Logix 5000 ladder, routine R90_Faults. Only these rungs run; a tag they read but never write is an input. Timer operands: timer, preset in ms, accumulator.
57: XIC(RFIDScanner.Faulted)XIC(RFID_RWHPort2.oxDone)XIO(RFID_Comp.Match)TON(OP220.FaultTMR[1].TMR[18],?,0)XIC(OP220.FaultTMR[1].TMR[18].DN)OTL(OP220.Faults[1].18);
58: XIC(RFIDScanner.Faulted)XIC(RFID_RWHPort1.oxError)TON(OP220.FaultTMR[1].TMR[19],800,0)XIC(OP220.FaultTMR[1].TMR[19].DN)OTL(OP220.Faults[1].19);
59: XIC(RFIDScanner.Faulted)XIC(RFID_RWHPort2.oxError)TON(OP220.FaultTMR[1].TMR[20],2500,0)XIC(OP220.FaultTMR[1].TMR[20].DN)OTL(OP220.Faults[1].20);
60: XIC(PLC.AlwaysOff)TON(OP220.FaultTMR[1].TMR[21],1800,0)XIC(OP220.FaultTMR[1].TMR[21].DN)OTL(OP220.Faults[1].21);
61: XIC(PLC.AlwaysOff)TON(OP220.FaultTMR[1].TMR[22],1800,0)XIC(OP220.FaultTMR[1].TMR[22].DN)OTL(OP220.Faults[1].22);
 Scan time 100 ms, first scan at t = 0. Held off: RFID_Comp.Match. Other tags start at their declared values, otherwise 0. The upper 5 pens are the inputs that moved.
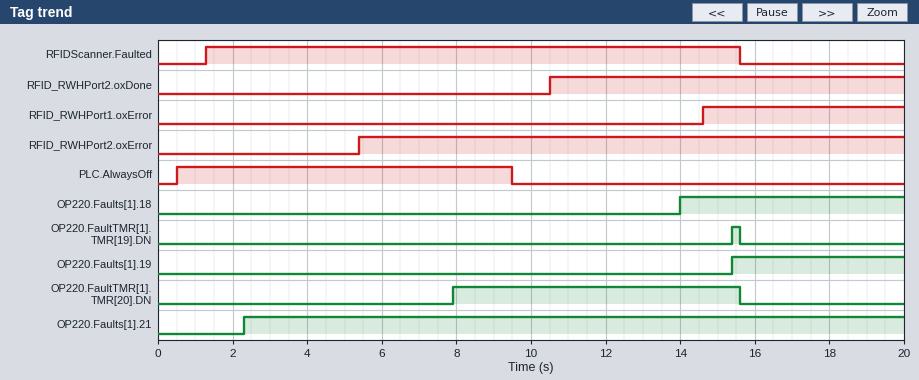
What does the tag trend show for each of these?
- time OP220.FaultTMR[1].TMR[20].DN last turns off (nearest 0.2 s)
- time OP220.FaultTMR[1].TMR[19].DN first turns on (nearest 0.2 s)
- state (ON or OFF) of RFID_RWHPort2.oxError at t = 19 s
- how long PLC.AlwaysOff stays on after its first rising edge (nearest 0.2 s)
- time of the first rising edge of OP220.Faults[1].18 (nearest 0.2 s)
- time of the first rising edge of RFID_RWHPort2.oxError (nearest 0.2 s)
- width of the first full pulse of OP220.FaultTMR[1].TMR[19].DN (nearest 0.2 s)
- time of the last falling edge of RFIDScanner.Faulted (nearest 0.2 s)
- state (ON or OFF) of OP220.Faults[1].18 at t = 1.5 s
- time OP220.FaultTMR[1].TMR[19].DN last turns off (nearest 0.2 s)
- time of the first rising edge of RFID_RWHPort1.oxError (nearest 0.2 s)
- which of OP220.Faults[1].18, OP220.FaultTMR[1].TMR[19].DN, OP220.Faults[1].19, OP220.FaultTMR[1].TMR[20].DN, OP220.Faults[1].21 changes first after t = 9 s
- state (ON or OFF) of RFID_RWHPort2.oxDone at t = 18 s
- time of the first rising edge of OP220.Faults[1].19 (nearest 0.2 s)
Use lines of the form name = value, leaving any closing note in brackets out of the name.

time OP220.FaultTMR[1].TMR[20].DN last turns off = 15.6 s
time OP220.FaultTMR[1].TMR[19].DN first turns on = 15.4 s
state (ON or OFF) of RFID_RWHPort2.oxError at t = 19 s = ON
how long PLC.AlwaysOff stays on after its first rising edge = 9.0 s
time of the first rising edge of OP220.Faults[1].18 = 14.0 s
time of the first rising edge of RFID_RWHPort2.oxError = 5.4 s
width of the first full pulse of OP220.FaultTMR[1].TMR[19].DN = 0.2 s
time of the last falling edge of RFIDScanner.Faulted = 15.6 s
state (ON or OFF) of OP220.Faults[1].18 at t = 1.5 s = OFF
time OP220.FaultTMR[1].TMR[19].DN last turns off = 15.6 s
time of the first rising edge of RFID_RWHPort1.oxError = 14.6 s
which of OP220.Faults[1].18, OP220.FaultTMR[1].TMR[19].DN, OP220.Faults[1].19, OP220.FaultTMR[1].TMR[20].DN, OP220.Faults[1].21 changes first after t = 9 s = OP220.Faults[1].18
state (ON or OFF) of RFID_RWHPort2.oxDone at t = 18 s = ON
time of the first rising edge of OP220.Faults[1].19 = 15.4 s
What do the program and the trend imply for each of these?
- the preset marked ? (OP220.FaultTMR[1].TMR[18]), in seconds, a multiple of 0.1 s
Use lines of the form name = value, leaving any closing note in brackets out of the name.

the preset marked ? (OP220.FaultTMR[1].TMR[18]), in seconds, a multiple of 0.1 s = 3.5 s
